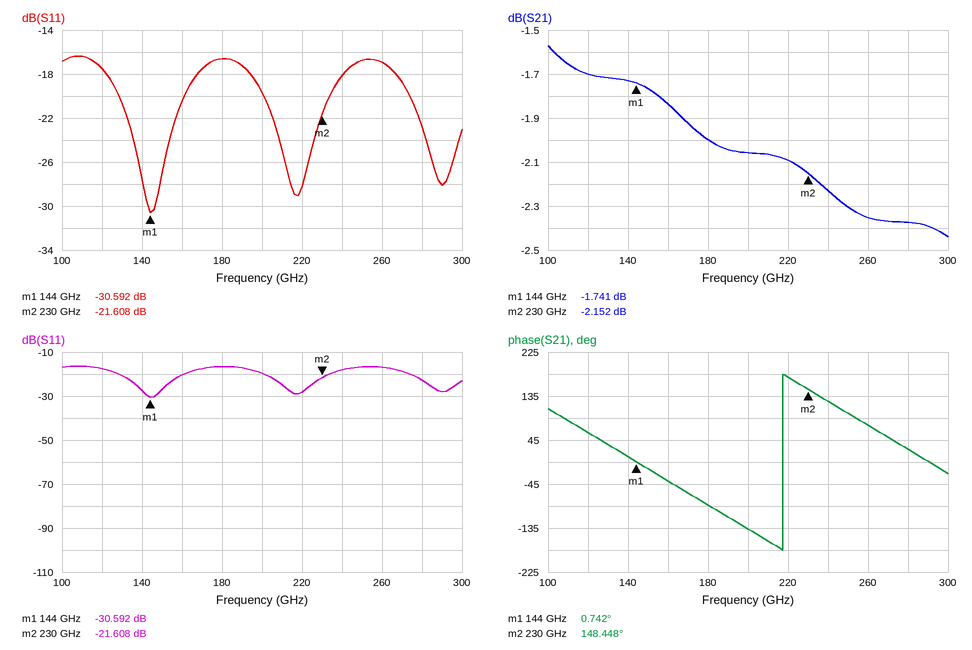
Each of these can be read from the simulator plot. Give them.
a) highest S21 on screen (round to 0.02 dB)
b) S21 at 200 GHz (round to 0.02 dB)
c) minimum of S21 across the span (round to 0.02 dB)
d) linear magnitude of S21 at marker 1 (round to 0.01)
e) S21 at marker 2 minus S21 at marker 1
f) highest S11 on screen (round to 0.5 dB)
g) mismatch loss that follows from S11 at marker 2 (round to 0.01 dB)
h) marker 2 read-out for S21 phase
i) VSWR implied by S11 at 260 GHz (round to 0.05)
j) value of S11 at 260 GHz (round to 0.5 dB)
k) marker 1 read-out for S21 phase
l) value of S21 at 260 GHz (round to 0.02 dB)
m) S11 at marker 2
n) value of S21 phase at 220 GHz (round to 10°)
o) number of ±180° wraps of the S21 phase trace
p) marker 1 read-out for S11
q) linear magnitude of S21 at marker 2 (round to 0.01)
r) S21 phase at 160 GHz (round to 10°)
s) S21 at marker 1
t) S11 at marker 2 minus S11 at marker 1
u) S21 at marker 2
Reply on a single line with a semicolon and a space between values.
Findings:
-1.58 dB; -2.06 dB; -2.44 dB; 0.82; -0.411 dB; -16.5 dB; 0.03 dB; 148.448°; 1.35; -17.0 dB; 0.742°; -2.36 dB; -21.608 dB; 170°; 1; -30.592 dB; 0.78; -40°; -1.741 dB; 8.984 dB; -2.152 dB
